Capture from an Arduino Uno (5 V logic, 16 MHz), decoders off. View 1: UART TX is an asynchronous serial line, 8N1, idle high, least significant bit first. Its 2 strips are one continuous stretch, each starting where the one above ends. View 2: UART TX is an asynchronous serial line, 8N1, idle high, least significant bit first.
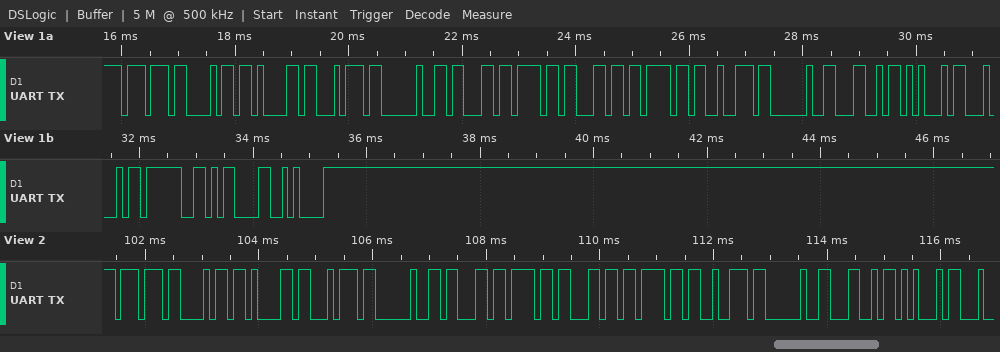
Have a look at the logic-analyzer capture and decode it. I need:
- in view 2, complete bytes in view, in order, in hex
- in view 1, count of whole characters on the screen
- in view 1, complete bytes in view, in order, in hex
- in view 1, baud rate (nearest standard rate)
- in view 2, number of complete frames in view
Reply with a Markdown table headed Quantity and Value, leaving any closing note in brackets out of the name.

| Quantity | Value |
|---|---|
| in view 2, complete bytes in view, in order, in hex | 77 68 61 74 20 63 6F 6C 6F 72 20 4C 45 |
| in view 1, count of whole characters on the screen | 17 |
| in view 1, complete bytes in view, in order, in hex | 77 68 61 74 20 63 6F 6C 6F 72 20 4C 45 44 3F 0D 0A |
| in view 1, baud rate | 9600 baud |
| in view 2, number of complete frames in view | 13 |
